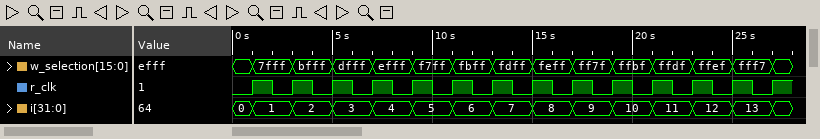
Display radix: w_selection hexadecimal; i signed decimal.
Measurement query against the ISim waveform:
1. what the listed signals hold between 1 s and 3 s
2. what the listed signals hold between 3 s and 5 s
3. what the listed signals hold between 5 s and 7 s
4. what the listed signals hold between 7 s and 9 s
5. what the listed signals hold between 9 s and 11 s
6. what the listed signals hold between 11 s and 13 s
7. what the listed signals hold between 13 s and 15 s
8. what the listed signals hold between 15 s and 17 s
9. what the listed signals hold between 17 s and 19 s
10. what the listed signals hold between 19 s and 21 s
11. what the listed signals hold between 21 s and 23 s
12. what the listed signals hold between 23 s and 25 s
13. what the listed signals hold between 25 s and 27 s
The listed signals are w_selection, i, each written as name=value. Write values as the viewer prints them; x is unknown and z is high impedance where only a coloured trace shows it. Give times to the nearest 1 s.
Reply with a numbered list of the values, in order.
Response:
1. w_selection=7fff, i=1
2. w_selection=bfff, i=2
3. w_selection=dfff, i=3
4. w_selection=efff, i=4
5. w_selection=f7ff, i=5
6. w_selection=fbff, i=6
7. w_selection=fdff, i=7
8. w_selection=feff, i=8
9. w_selection=ff7f, i=9
10. w_selection=ffbf, i=10
11. w_selection=ffdf, i=11
12. w_selection=ffef, i=12
13. w_selection=fff7, i=13
